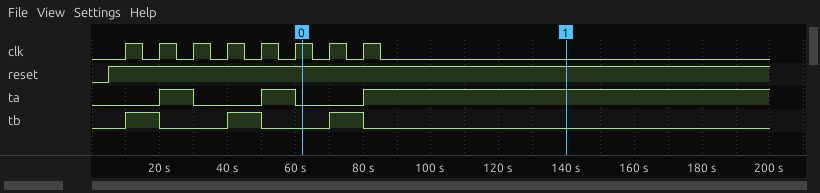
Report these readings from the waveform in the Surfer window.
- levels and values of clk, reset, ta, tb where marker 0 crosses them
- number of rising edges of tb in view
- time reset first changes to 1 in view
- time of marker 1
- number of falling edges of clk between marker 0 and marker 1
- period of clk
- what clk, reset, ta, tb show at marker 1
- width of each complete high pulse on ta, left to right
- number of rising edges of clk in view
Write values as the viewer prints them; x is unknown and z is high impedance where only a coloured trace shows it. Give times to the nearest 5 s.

clk=1, reset=1, ta=0, tb=0
3
5 s
140 s
3
10 s
clk=0, reset=1, ta=1, tb=0
10 s, 10 s
8
